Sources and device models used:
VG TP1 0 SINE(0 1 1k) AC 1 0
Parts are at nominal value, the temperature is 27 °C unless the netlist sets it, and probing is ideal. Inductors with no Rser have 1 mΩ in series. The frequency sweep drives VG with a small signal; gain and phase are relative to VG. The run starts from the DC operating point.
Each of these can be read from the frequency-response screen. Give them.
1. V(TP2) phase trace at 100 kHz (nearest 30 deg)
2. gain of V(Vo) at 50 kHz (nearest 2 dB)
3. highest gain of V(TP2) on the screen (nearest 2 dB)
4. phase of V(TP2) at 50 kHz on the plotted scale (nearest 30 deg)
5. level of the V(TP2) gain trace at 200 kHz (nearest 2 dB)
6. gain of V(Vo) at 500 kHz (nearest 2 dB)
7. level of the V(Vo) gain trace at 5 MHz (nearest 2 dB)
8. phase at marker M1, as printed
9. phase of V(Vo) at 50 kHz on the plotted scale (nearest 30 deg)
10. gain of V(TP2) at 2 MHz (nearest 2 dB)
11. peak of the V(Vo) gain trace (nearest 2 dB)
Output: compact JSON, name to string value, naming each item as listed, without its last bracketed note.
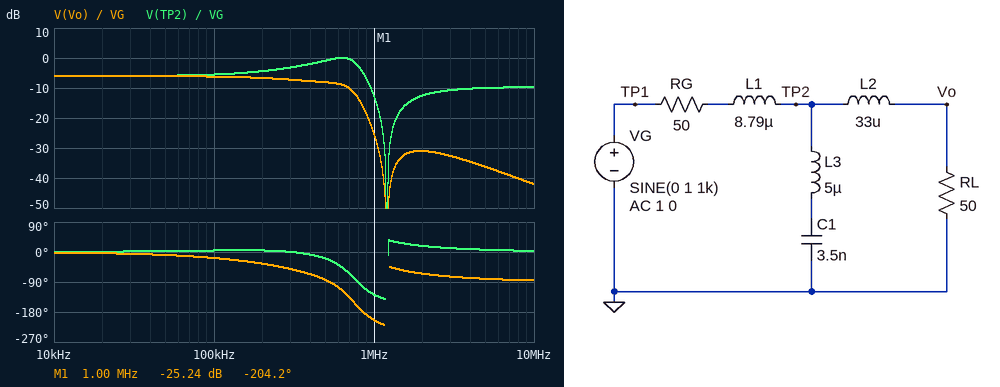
{"V(TP2) phase trace at 100 kHz": "0 deg", "gain of V(Vo) at 50 kHz": "-6 dB", "highest gain of V(TP2) on the screen": "0 dB", "phase of V(TP2) at 50 kHz on the plotted scale": "0 deg", "level of the V(TP2) gain trace at 200 kHz": "-4 dB", "gain of V(Vo) at 500 kHz": "-8 dB", "level of the V(Vo) gain trace at 5 MHz": "-36 dB", "phase at marker M1, as printed": "-204.2 deg", "phase of V(Vo) at 50 kHz on the plotted scale": "0 deg", "gain of V(TP2) at 2 MHz": "-12 dB", "peak of the V(Vo) gain trace": "-6 dB"}
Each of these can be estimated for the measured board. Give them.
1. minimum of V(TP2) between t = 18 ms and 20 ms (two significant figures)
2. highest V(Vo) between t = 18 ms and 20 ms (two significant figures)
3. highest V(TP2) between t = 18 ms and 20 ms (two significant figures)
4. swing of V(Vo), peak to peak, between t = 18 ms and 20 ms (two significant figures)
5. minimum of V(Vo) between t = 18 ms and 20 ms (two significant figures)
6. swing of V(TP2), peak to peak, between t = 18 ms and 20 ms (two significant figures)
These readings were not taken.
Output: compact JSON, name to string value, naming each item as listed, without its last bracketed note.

{"minimum of V(TP2) between t = 18 ms and 20 ms": "-500 mV", "highest V(Vo) between t = 18 ms and 20 ms": "500 mV", "highest V(TP2) between t = 18 ms and 20 ms": "500 mV", "swing of V(Vo), peak to peak, between t = 18 ms and 20 ms": "1.0 V", "minimum of V(Vo) between t = 18 ms and 20 ms": "-500 mV", "swing of V(TP2), peak to peak, between t = 18 ms and 20 ms": "1.0 V"}
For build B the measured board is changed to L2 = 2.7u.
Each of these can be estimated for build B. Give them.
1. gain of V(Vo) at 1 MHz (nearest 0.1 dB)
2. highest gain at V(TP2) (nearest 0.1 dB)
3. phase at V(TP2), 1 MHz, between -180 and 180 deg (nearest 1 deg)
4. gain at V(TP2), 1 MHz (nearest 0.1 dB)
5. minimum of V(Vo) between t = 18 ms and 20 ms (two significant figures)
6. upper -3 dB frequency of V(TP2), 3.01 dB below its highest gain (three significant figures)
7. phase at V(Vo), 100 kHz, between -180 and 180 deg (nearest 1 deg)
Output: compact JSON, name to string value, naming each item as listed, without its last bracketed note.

{"gain of V(Vo) at 1 MHz": "-13.7 dB", "highest gain at V(TP2)": "-6.0 dB", "phase at V(TP2), 1 MHz, between -180 and 180 deg": "-112 deg", "gain at V(TP2), 1 MHz": "-13.2 dB", "minimum of V(Vo) between t = 18 ms and 20 ms": "-500 mV", "upper -3 dB frequency of V(TP2), 3.01 dB below its highest gain": "893 kHz", "phase at V(Vo), 100 kHz, between -180 and 180 deg": "-7 deg"}
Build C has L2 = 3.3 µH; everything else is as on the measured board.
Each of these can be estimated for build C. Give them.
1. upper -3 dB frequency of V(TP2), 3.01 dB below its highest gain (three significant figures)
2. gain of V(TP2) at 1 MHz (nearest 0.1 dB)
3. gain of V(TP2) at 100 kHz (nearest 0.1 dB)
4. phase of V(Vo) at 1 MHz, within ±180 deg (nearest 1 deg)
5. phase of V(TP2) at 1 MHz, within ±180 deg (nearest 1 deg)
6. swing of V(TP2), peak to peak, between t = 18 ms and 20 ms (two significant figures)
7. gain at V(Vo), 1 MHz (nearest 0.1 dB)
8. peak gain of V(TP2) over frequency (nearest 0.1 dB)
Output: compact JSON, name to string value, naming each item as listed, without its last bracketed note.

{"upper -3 dB frequency of V(TP2), 3.01 dB below its highest gain": "899 kHz", "gain of V(TP2) at 1 MHz": "-13.0 dB", "gain of V(TP2) at 100 kHz": "-6.0 dB", "phase of V(Vo) at 1 MHz, within ±180 deg": "-135 deg", "phase of V(TP2) at 1 MHz, within ±180 deg": "-112 deg", "swing of V(TP2), peak to peak, between t = 18 ms and 20 ms": "1.0 V", "gain at V(Vo), 1 MHz": "-13.7 dB", "peak gain of V(TP2) over frequency": "-5.9 dB"}
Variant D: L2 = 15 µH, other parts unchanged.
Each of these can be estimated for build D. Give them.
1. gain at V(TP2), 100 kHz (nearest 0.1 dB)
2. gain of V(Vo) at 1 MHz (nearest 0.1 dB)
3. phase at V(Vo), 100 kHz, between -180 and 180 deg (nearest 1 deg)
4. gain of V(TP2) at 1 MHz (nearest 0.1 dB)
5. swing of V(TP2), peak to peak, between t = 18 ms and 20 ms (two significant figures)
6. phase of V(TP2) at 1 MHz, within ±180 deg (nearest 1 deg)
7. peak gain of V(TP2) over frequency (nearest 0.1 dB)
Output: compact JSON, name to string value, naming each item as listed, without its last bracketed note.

{"gain at V(TP2), 100 kHz": "-5.9 dB", "gain of V(Vo) at 1 MHz": "-18.8 dB", "phase at V(Vo), 100 kHz, between -180 and 180 deg": "-12 deg", "gain of V(TP2) at 1 MHz": "-12.2 dB", "swing of V(TP2), peak to peak, between t = 18 ms and 20 ms": "1.0 V", "phase of V(TP2) at 1 MHz, within ±180 deg": "-124 deg", "peak gain of V(TP2) over frequency": "-2.1 dB"}
